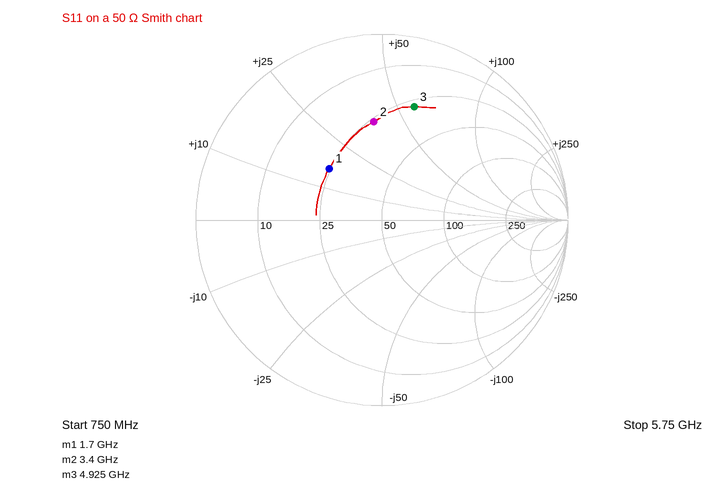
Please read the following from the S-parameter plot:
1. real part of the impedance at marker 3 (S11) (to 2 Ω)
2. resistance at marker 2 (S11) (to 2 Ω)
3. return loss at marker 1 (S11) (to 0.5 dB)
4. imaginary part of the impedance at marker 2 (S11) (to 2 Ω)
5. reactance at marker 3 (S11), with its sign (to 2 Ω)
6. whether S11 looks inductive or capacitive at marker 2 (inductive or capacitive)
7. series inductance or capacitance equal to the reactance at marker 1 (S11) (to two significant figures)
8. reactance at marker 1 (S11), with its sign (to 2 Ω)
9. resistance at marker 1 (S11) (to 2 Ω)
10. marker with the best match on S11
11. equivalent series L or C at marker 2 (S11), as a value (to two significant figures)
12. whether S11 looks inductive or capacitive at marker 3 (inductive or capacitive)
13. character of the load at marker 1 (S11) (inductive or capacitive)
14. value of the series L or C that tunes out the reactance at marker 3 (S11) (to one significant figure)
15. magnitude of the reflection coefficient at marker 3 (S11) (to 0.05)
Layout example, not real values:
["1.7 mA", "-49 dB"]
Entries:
["28 Ω", "26 Ω", "8.0 dB", "+38 Ω", "+58 Ω", "inductive", "1.5 nH", "+16 Ω", "24 Ω", "marker 1", "1.8 nH", "inductive", "inductive", "600 fF", "0.65"]
